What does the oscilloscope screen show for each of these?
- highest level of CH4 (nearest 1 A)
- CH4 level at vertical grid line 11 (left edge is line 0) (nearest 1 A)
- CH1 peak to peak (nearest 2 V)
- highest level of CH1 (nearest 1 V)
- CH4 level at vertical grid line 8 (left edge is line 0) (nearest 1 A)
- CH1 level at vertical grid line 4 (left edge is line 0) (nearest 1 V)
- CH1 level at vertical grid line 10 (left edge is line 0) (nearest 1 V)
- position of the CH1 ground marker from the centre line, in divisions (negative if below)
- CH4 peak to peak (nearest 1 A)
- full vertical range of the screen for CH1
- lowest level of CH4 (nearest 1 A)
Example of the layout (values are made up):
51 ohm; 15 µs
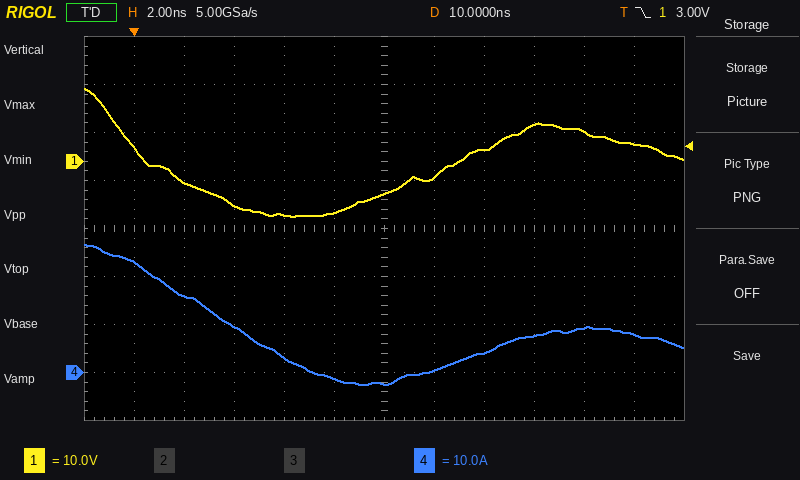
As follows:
27 A; 8 A; 26 V; 15 V; 4 A; -11 V; 6 V; +1.4 div; 29 A; 80 V; -2 A
